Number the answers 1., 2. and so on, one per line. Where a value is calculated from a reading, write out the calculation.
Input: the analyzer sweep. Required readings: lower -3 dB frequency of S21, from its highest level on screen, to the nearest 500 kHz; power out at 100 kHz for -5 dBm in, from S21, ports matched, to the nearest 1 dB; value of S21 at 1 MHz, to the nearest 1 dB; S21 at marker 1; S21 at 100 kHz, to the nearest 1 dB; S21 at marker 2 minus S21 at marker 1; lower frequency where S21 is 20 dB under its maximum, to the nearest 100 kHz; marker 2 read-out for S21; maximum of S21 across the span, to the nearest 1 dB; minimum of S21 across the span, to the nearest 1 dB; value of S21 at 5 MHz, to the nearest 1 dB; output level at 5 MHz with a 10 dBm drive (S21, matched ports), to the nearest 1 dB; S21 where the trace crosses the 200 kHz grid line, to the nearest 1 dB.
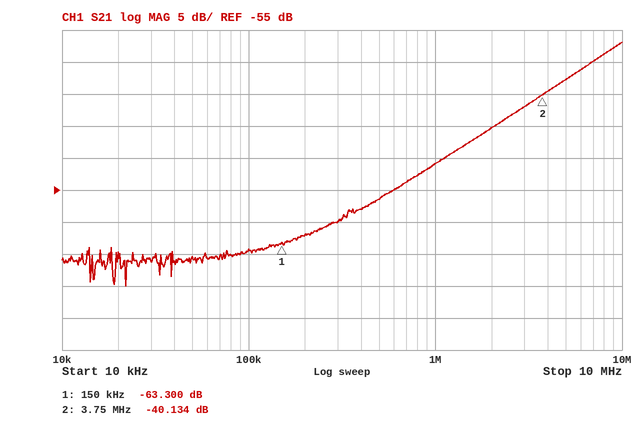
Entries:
1. 7.0 MHz
2. -5 dBm + (-64 dB) = -69 dBm
3. -51 dB
4. -63.300 dB
5. -64 dB
6. -40.134 − (-63.3) = 23.166 dB
7. 900 kHz
8. -40.134 dB
9. -32 dB
10. -70 dB
11. -38 dB
12. 10 dBm + (-38 dB) = -28 dBm
13. -62 dB
